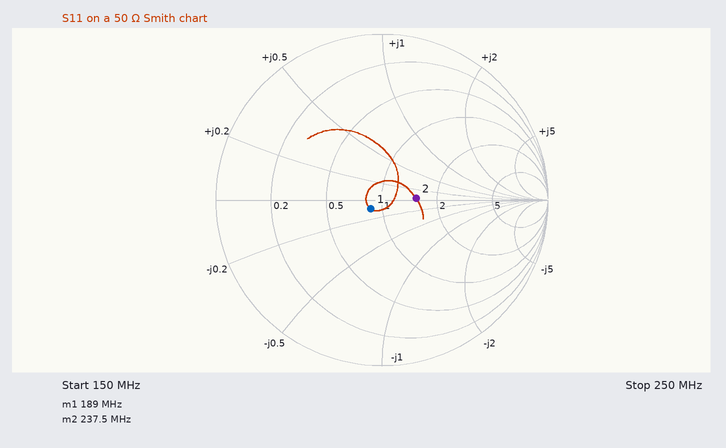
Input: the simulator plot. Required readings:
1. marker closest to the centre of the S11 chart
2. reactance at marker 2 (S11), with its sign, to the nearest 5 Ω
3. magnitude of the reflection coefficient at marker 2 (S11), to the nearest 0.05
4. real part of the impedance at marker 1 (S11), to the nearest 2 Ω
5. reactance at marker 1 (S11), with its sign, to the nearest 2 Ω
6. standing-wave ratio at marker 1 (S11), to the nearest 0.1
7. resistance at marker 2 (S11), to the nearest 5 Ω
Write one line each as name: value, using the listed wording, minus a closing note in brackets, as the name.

marker closest to the centre of the S11 chart: marker 1
reactance at marker 2 (S11), with its sign, to the nearest 5 Ω: 0 Ω
magnitude of the reflection coefficient at marker 2 (S11), to the nearest 0.05: 0.20
real part of the impedance at marker 1 (S11), to the nearest 2 Ω: 44 Ω
reactance at marker 1 (S11), with its sign, to the nearest 2 Ω: -4 Ω
standing-wave ratio at marker 1 (S11), to the nearest 0.1: 1.2
resistance at marker 2 (S11), to the nearest 5 Ω: 75 Ω
